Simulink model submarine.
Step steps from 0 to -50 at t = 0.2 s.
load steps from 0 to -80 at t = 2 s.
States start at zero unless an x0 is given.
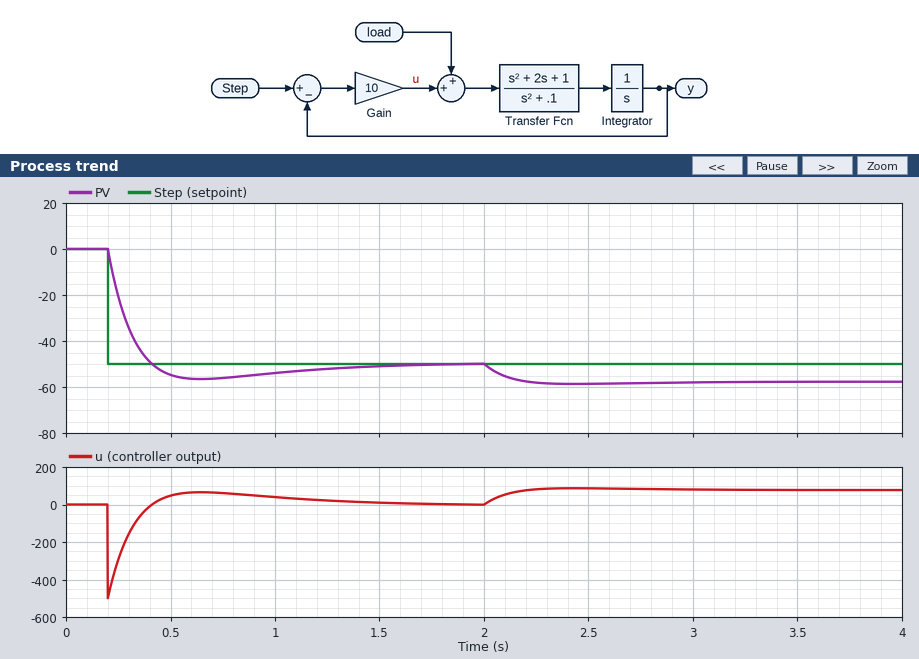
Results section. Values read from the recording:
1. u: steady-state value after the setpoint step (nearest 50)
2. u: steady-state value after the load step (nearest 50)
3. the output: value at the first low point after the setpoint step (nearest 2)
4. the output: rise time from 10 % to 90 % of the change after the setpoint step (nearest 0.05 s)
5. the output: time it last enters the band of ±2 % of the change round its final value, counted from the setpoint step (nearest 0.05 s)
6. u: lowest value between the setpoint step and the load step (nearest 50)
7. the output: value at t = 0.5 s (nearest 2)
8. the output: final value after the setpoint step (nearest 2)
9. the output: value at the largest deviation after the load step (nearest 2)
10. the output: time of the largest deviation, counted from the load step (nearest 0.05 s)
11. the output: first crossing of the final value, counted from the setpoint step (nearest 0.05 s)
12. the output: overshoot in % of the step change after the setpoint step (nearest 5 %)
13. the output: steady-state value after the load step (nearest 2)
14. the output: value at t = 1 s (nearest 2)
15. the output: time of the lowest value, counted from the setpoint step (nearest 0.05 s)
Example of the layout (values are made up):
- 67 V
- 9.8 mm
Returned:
- 0
- 100
- -56
- 0.15 s
- 1.30 s
- -500
- -54
- -50
- -58
- 0.45 s
- 0.20 s
- 15 %
- -58
- -54
- 0.45 s
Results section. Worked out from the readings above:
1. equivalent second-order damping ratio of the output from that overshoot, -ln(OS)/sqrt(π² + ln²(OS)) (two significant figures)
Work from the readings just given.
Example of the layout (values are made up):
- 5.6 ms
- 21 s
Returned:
- 0.52
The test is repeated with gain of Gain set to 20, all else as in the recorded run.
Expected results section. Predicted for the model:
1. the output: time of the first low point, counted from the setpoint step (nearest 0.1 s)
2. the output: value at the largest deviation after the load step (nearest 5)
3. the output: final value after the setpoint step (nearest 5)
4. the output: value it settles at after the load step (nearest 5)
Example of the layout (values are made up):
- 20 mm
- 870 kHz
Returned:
- 0.3 s
- -55
- -50
- -55
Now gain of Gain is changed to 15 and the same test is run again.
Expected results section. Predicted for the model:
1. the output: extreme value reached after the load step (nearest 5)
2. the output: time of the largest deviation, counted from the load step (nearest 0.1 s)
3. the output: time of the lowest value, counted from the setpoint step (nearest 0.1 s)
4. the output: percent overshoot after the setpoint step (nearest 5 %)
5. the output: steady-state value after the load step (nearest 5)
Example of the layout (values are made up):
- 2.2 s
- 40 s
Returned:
- -55
- 0.3 s
- 0.3 s
- 10 %
- -55
